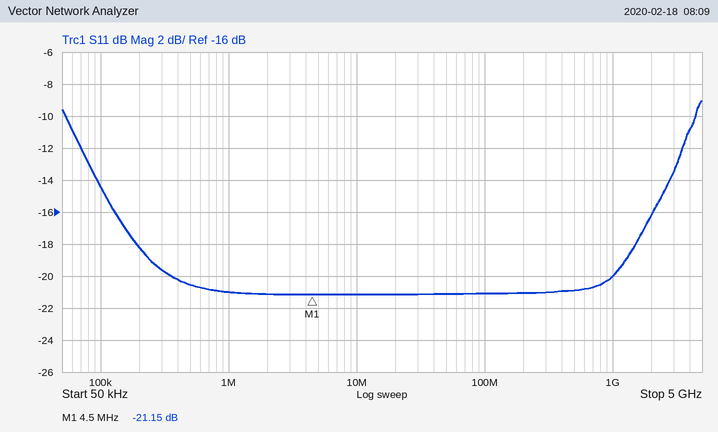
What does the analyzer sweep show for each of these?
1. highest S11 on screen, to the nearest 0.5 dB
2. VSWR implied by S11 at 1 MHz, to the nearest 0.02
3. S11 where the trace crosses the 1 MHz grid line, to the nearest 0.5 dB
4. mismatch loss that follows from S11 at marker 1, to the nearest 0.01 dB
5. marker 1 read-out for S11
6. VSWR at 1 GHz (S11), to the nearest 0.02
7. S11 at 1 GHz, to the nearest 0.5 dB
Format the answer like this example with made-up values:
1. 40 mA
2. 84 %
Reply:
1. -9.0 dB
2. 1.20
3. -21.0 dB
4. 0.03 dB
5. -21.15 dB
6. 1.22
7. -20.0 dB
